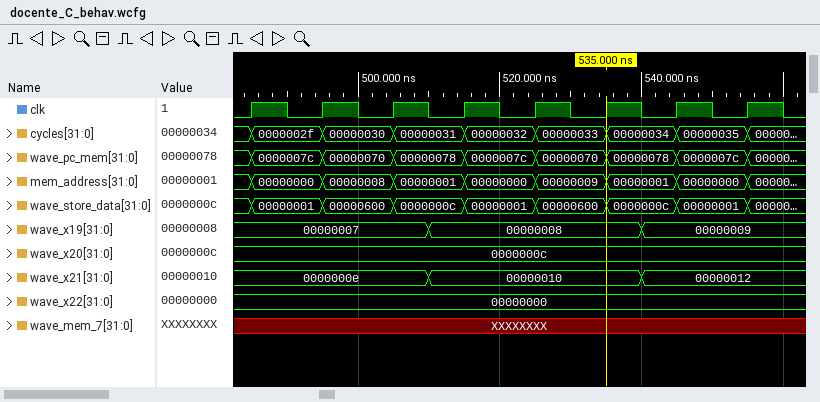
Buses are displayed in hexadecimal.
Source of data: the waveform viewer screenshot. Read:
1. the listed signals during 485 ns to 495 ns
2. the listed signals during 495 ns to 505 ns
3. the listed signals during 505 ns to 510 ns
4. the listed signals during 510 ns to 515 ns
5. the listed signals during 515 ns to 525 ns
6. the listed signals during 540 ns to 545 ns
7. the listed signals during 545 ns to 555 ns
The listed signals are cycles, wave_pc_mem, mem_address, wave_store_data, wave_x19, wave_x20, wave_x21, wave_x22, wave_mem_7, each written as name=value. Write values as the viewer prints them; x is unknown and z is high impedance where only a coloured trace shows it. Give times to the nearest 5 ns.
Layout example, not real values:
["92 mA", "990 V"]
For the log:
["cycles=0000002f, wave_pc_mem=0000007c, mem_address=00000000, wave_store_data=00000001, wave_x19=00000007, wave_x20=0000000c, wave_x21=0000000e, wave_x22=00000000, wave_mem_7=XXXXXXXX", "cycles=00000030, wave_pc_mem=00000070, mem_address=00000008, wave_store_data=00000600, wave_x19=00000007, wave_x20=0000000c, wave_x21=0000000e, wave_x22=00000000, wave_mem_7=XXXXXXXX", "cycles=00000031, wave_pc_mem=00000078, mem_address=00000001, wave_store_data=0000000c, wave_x19=00000007, wave_x20=0000000c, wave_x21=0000000e, wave_x22=00000000, wave_mem_7=XXXXXXXX", "cycles=00000031, wave_pc_mem=00000078, mem_address=00000001, wave_store_data=0000000c, wave_x19=00000008, wave_x20=0000000c, wave_x21=00000010, wave_x22=00000000, wave_mem_7=XXXXXXXX", "cycles=00000032, wave_pc_mem=0000007c, mem_address=00000000, wave_store_data=00000001, wave_x19=00000008, wave_x20=0000000c, wave_x21=00000010, wave_x22=00000000, wave_mem_7=XXXXXXXX", "cycles=00000034, wave_pc_mem=00000078, mem_address=00000001, wave_store_data=0000000c, wave_x19=00000009, wave_x20=0000000c, wave_x21=00000012, wave_x22=00000000, wave_mem_7=XXXXXXXX", "cycles=00000035, wave_pc_mem=0000007c, mem_address=00000000, wave_store_data=00000001, wave_x19=00000009, wave_x20=0000000c, wave_x21=00000012, wave_x22=00000000, wave_mem_7=XXXXXXXX"]
